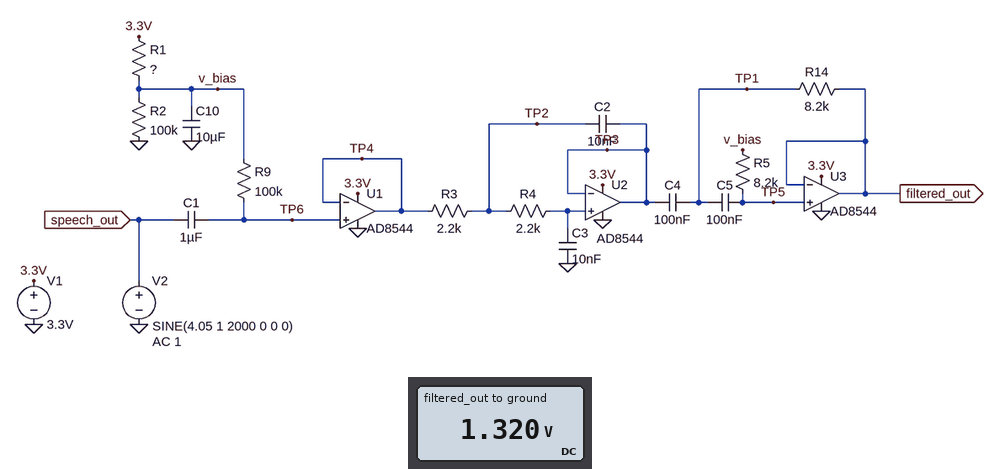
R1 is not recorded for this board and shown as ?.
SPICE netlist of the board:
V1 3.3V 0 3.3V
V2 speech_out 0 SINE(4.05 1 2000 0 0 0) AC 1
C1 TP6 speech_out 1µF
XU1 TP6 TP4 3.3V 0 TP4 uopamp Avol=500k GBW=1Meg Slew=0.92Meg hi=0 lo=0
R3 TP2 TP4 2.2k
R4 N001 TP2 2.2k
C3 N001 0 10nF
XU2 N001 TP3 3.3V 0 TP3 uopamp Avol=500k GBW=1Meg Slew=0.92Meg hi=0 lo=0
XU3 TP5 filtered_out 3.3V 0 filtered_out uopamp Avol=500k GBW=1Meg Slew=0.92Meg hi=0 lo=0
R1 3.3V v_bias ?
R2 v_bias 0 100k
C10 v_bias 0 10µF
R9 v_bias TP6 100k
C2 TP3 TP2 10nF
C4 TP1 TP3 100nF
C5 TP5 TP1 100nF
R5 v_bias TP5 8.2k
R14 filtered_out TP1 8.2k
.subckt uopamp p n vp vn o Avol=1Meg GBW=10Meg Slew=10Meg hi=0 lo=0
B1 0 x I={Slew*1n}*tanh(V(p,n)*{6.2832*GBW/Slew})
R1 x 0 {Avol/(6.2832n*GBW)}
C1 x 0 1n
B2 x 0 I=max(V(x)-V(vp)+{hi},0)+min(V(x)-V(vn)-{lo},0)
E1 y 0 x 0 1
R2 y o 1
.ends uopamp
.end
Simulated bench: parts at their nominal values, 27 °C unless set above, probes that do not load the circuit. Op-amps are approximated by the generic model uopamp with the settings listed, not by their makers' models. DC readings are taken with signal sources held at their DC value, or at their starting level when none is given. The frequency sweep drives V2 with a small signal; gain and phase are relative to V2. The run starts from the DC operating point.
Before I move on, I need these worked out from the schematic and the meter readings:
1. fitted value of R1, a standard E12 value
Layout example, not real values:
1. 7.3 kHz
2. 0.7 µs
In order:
1. 150 kΩ
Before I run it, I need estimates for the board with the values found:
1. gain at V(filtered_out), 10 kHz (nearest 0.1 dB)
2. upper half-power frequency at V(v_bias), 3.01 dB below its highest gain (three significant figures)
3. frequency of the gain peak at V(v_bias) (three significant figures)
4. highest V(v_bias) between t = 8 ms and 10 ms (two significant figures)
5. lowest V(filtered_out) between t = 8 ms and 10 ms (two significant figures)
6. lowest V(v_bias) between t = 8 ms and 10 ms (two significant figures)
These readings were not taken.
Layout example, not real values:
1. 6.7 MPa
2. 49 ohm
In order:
1. -9.3 dB
2. 2.20 Hz
3. 649 mHz
4. 1.3 V
5. 400 mV
6. 1.3 V
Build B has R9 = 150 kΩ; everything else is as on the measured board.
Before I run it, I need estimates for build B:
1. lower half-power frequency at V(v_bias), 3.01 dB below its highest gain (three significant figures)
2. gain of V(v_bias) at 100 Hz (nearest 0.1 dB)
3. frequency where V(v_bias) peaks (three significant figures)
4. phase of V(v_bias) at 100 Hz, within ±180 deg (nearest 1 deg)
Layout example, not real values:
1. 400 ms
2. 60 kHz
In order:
1. 175 mHz
2. -48.9 dB
3. 530 mHz
4. 20 deg
